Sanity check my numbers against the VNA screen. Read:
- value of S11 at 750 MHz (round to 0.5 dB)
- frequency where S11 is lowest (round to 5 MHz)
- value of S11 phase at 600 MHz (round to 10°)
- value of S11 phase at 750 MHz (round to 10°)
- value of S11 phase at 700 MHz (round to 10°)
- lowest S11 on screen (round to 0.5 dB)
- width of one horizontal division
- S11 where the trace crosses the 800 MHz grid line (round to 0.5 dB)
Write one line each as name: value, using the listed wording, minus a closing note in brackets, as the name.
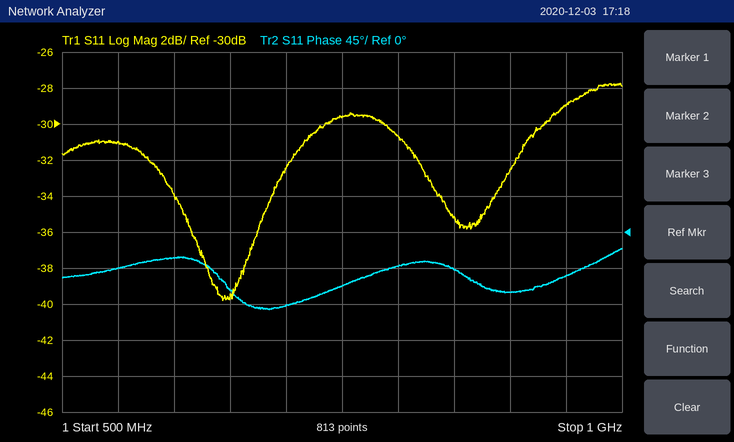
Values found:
value of S11 at 750 MHz: -29.5 dB
frequency where S11 is lowest: 645 MHz
value of S11 phase at 600 MHz: -30°
value of S11 phase at 750 MHz: -70°
value of S11 phase at 700 MHz: -90°
lowest S11 on screen: -40.0 dB
width of one horizontal division: 50 MHz
S11 where the trace crosses the 800 MHz grid line: -30.5 dB
